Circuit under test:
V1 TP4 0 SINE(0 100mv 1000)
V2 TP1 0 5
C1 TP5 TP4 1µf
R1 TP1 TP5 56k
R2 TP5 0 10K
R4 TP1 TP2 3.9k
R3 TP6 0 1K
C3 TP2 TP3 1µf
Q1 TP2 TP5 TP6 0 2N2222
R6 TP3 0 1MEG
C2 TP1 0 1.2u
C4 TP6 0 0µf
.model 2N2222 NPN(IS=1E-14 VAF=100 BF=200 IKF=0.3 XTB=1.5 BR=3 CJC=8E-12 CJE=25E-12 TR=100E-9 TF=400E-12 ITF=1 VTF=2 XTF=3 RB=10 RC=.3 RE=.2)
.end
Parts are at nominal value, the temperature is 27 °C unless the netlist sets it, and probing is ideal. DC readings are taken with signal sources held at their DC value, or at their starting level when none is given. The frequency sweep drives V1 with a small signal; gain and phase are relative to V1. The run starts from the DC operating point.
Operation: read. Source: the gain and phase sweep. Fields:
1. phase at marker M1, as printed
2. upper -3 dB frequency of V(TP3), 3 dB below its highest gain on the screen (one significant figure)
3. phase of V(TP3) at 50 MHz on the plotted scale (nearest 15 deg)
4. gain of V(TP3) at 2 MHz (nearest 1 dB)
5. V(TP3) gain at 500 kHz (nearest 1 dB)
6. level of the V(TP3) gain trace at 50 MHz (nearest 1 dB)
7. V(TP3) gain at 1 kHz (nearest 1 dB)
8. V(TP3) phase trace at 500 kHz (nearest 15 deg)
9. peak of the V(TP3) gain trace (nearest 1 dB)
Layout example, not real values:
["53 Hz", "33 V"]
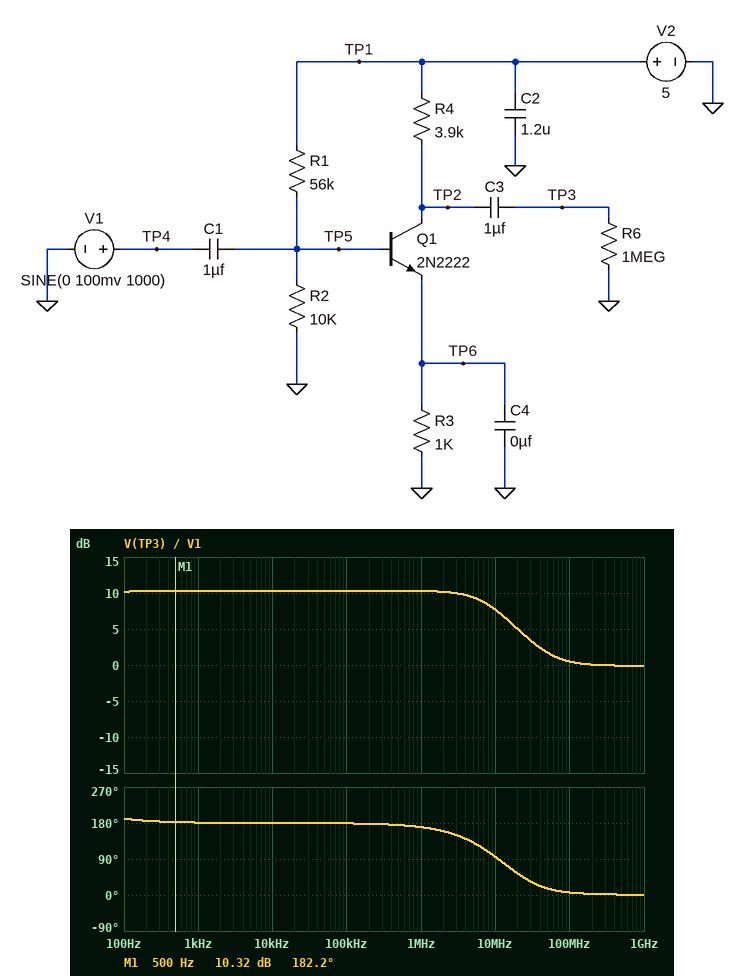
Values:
["182.2 deg", "10 MHz", "15 deg", "10 dB", "10 dB", "2 dB", "10 dB", "180 deg", "10 dB"]
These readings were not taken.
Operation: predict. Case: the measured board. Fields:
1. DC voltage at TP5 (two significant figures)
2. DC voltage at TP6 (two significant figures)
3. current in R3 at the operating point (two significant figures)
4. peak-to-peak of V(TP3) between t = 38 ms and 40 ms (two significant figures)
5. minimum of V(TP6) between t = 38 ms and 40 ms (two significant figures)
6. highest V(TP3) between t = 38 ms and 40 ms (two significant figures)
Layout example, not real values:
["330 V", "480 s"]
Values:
["750 mV", "150 mV", "150 µA", "650 mV", "67 mV", "310 mV"]
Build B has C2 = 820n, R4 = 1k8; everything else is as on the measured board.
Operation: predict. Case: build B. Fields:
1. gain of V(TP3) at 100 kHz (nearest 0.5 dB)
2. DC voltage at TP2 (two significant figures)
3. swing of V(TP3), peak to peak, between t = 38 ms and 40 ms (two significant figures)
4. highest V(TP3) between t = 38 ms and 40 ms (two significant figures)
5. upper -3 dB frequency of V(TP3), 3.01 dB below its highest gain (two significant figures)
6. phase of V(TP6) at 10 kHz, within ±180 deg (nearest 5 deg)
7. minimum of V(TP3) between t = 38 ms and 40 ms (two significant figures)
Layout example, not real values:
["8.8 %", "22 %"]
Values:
["3.5 dB", "4.7 V", "300 mV", "140 mV", "75 MHz", "0 deg", "-160 mV"]
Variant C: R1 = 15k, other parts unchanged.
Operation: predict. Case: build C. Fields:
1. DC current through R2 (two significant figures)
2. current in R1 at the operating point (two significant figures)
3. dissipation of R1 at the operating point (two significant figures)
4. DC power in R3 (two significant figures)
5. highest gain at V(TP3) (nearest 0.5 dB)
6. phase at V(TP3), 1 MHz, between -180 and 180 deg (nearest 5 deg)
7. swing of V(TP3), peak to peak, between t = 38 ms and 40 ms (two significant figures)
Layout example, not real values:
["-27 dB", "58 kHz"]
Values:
["170 µA", "220 µA", "720 µW", "1.1 mW", "0 dB", "20 deg", "270 mV"]
